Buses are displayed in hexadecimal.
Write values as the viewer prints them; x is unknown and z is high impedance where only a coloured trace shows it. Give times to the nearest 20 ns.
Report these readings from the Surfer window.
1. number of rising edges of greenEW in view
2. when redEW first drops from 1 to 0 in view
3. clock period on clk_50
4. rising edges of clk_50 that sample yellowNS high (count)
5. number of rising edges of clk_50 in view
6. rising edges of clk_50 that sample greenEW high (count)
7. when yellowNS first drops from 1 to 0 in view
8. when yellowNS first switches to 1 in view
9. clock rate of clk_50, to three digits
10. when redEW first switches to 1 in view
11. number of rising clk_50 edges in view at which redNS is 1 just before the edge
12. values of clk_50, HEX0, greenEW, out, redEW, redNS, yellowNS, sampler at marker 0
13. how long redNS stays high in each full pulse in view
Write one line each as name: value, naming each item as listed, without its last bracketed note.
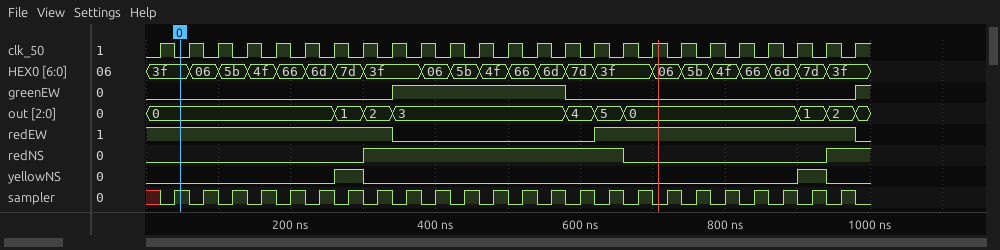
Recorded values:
number of rising edges of greenEW in view: 2
when redEW first drops from 1 to 0 in view: 340 ns
clock period on clk_50: 40 ns
rising edges of clk_50 that sample yellowNS high: 2
number of rising edges of clk_50 in view: 25
rising edges of clk_50 that sample greenEW high: 6
when yellowNS first drops from 1 to 0 in view: 300 ns
when yellowNS first switches to 1 in view: 260 ns
clock rate of clk_50, to three digits: 25.0 MHz
when redEW first switches to 1 in view: 620 ns
number of rising clk_50 edges in view at which redNS is 1 just before the edge: 10
values of clk_50, HEX0, greenEW, out, redEW, redNS, yellowNS, sampler at marker 0: clk_50=0, HEX0=3f, greenEW=0, out=0, redEW=1, redNS=0, yellowNS=0, sampler=1
how long redNS stays high in each full pulse in view: 360 ns
